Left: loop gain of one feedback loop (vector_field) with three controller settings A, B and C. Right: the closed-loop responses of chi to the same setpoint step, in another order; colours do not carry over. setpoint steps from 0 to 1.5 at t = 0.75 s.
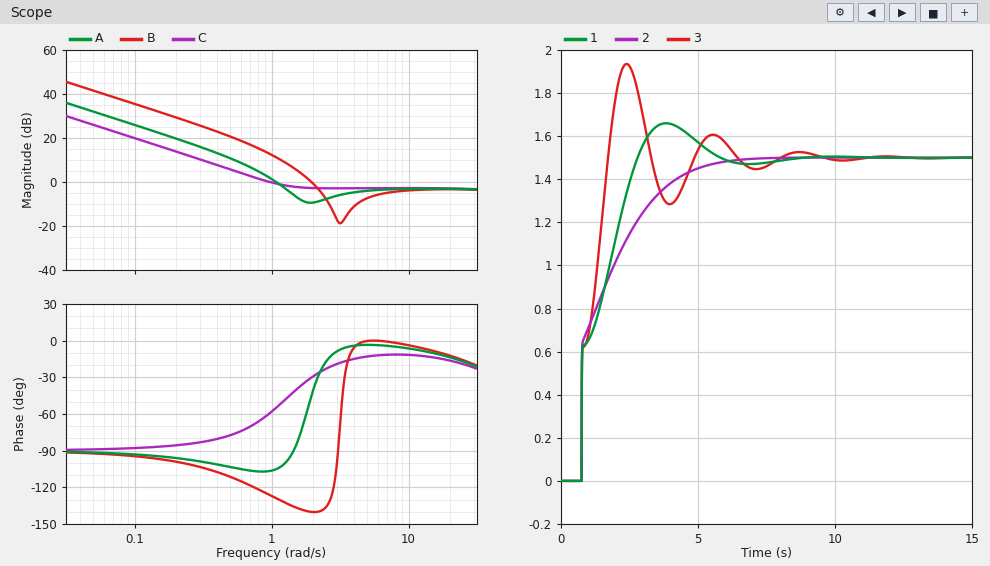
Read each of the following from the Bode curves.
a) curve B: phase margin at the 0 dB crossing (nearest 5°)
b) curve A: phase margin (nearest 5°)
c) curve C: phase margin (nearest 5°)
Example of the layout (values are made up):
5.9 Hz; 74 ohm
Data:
40°; 75°; 120°
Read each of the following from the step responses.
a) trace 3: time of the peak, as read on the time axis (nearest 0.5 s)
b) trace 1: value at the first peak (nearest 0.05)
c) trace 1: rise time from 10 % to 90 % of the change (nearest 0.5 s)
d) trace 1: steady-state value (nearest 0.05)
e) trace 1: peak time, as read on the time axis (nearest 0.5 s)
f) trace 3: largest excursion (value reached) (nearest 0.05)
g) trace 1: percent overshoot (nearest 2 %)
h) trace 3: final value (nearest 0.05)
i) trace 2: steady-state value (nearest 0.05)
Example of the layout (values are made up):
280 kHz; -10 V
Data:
2.5 s; 1.65; 1.5 s; 1.50; 4.0 s; 1.95; 10 %; 1.50; 1.50
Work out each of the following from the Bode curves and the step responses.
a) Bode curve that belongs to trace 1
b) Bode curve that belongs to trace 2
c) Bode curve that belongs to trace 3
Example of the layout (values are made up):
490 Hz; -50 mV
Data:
A; C; B
